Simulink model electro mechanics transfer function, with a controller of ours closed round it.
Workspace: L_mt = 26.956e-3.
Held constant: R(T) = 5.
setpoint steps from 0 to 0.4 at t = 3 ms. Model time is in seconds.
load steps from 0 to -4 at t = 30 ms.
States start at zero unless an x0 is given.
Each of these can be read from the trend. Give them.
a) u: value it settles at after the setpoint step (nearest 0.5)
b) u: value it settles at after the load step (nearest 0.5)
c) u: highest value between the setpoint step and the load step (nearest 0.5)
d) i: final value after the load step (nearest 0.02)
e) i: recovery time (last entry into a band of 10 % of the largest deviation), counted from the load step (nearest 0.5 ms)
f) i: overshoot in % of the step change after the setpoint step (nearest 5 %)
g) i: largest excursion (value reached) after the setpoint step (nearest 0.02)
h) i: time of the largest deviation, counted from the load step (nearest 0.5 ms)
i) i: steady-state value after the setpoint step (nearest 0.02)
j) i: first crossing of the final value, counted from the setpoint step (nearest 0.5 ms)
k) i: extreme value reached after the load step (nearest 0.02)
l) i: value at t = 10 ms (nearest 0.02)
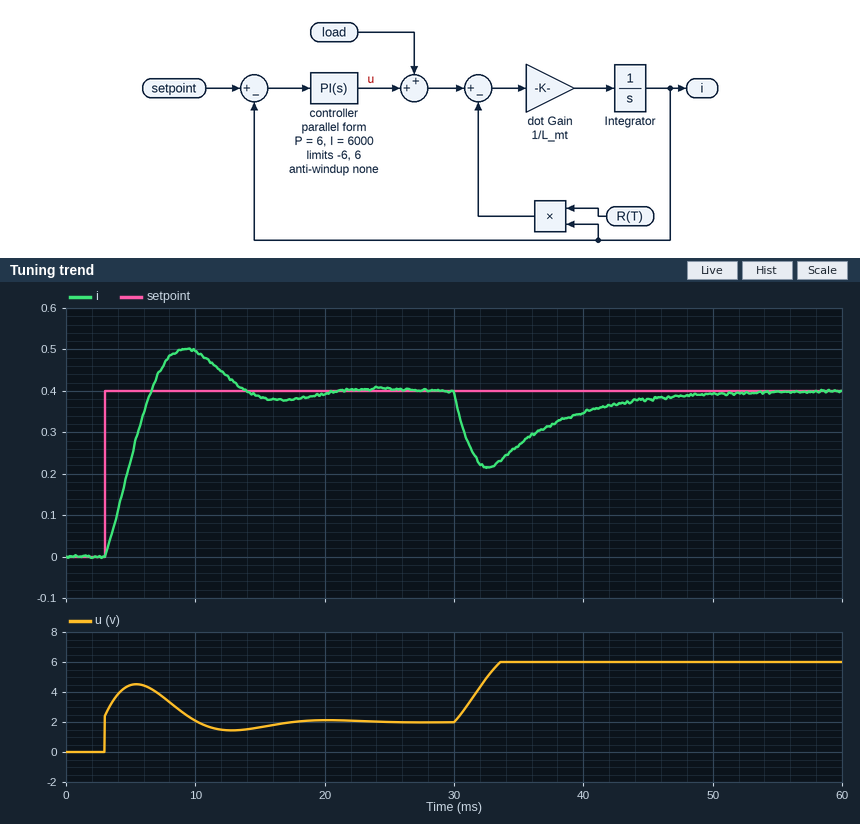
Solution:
2.0
6.0
4.5
0.40
15.5 ms
25 %
0.50
2.5 ms
0.40
3.5 ms
0.22
0.50
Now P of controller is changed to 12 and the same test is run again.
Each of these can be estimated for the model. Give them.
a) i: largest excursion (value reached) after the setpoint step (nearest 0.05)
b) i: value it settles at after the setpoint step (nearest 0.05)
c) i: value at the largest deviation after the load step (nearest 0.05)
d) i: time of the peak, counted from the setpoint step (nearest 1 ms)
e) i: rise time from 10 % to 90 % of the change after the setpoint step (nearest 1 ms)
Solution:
0.45
0.40
0.25
6 ms
3 ms
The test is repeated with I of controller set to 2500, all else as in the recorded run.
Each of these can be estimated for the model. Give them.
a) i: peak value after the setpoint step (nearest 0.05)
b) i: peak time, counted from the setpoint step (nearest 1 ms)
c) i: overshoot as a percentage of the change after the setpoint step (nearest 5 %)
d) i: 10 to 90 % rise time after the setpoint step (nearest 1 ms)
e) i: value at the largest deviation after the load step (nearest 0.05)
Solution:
0.45
10 ms
10 %
5 ms
0.15
